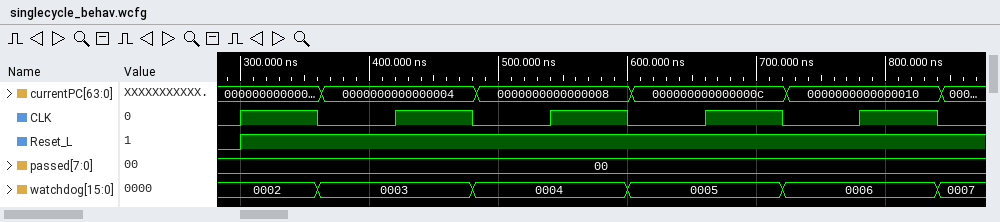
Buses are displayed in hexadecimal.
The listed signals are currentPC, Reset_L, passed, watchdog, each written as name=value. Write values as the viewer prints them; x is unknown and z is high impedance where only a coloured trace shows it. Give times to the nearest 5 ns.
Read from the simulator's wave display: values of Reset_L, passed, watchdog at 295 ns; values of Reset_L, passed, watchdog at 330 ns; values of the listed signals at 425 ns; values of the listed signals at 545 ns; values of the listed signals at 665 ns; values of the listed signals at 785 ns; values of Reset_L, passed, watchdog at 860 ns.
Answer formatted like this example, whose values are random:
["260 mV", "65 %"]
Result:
["Reset_L=0, passed=00, watchdog=0002", "Reset_L=1, passed=00, watchdog=0002", "currentPC=0000000000000004, Reset_L=1, passed=00, watchdog=0003", "currentPC=0000000000000008, Reset_L=1, passed=00, watchdog=0004", "currentPC=000000000000000c, Reset_L=1, passed=00, watchdog=0005", "currentPC=0000000000000010, Reset_L=1, passed=00, watchdog=0006", "Reset_L=1, passed=00, watchdog=0007"]
